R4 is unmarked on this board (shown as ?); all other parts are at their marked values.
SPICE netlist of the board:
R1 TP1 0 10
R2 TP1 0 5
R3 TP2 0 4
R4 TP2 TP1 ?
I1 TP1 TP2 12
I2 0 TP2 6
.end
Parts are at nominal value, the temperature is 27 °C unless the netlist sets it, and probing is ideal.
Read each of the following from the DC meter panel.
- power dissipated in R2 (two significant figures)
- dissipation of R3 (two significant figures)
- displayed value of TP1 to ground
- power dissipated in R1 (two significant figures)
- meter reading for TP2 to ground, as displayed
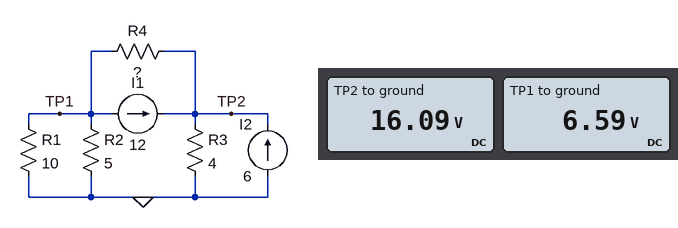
8.7 W
65 W
6.59 V
4.3 W
16.09 V
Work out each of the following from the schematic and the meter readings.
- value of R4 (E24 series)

0.68 Ω
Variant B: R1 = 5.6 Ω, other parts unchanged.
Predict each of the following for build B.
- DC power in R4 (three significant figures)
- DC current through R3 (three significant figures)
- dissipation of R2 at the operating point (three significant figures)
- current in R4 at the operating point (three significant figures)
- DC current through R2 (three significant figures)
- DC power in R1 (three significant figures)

136 W
3.84 A
6.53 W
14.2 A
1.14 A
5.83 W
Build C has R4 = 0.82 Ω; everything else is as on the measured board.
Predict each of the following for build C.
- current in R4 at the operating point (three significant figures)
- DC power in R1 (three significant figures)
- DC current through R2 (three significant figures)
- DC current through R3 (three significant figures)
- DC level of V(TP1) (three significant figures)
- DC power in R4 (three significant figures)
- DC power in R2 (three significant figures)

13.7 A
3.35 W
1.16 A
4.26 A
5.79 V
155 W
6.70 W
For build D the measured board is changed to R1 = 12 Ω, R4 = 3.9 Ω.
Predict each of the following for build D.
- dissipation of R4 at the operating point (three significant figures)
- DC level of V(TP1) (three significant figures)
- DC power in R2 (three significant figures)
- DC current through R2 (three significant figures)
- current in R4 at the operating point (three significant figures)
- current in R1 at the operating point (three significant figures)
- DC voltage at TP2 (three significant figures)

390 W
-7.04 V
9.91 W
1.41 A
10.0 A
587 mA
32.0 V
